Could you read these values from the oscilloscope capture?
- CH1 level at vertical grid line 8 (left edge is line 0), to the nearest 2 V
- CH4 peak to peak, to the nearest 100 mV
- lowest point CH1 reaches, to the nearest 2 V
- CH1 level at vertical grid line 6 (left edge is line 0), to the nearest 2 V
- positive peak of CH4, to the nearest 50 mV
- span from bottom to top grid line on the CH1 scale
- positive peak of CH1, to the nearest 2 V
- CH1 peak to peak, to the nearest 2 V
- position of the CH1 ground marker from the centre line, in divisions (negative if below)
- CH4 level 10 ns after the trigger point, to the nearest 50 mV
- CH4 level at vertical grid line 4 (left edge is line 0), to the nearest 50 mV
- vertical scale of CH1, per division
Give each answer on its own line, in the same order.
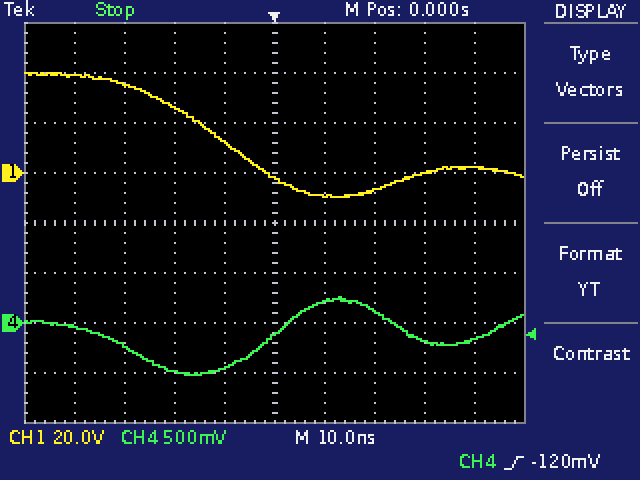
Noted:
0 V
800 mV
-10 V
-10 V
250 mV
160 V
40 V
50 V
+1.0 div
200 mV
-450 mV
20 V
